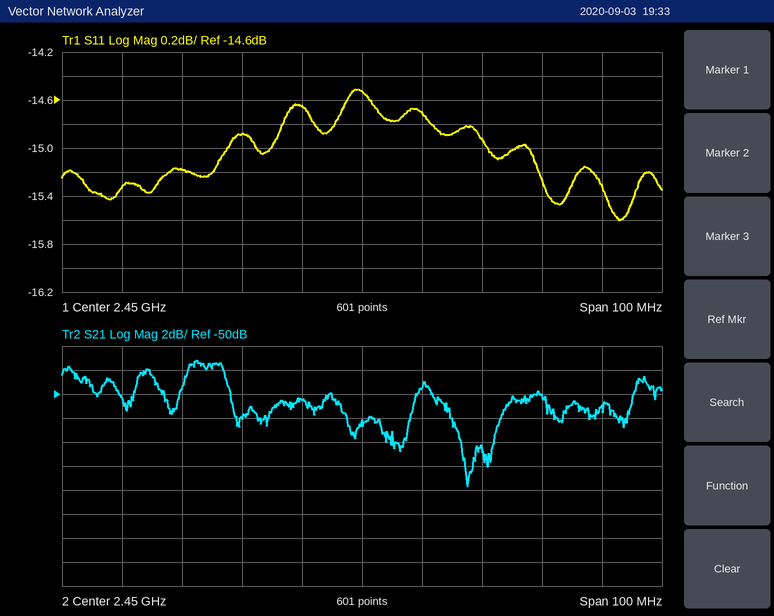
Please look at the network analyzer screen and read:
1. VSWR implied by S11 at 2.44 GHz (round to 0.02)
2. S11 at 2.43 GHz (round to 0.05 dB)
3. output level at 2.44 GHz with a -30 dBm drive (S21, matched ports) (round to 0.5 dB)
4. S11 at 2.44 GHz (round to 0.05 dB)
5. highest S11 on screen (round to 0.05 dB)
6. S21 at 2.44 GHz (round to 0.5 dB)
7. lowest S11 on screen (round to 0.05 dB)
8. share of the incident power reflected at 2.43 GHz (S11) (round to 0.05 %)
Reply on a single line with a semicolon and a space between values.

1.46; -14.90 dB; -80.5 dBm; -14.65 dB; -14.50 dB; -50.5 dB; -15.60 dB; 3.25 %
